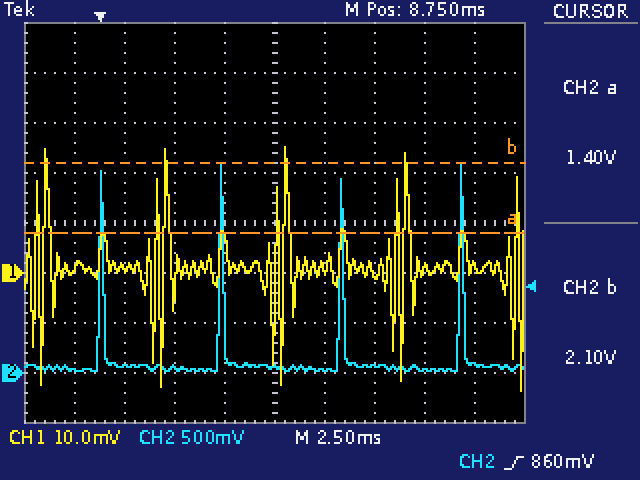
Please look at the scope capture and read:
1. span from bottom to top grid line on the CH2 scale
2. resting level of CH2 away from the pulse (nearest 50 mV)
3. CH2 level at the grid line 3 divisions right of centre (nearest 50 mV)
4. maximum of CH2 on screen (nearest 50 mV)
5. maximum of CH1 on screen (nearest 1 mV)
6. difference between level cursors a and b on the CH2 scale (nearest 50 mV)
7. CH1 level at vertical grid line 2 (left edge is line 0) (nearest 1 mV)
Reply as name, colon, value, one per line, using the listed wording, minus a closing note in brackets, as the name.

span from bottom to top grid line on the CH2 scale: 4 V
resting level of CH2 away from the pulse: 50 mV
CH2 level at the grid line 3 divisions right of centre: 50 mV
maximum of CH2 on screen: 2.10 V
maximum of CH1 on screen: 25 mV
difference between level cursors a and b on the CH2 scale: 700 mV
CH1 level at vertical grid line 2 (left edge is line 0): 1 mV
